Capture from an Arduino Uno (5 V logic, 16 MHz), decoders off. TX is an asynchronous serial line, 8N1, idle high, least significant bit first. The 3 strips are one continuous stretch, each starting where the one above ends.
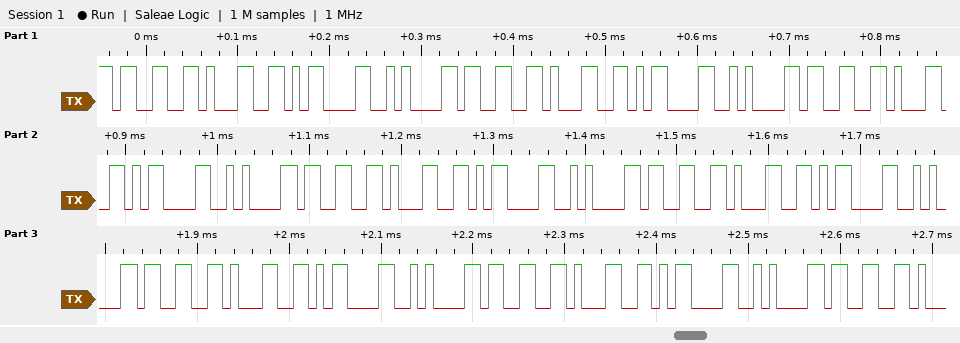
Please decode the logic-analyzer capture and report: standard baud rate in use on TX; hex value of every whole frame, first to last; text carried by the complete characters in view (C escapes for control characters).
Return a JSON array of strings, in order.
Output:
["115200 baud", "33 31 0D 0A 33 31 0D 0A 33 31 0D 0A 33 31 0D 0A 33 31 0D 0A 33 31 0D 0A 33 31 0D 0A 33", "\"31\\r\\n31\\r\\n31\\r\\n31\\r\\n31\\r\\n31\\r\\n31\\r\\n3\""]
